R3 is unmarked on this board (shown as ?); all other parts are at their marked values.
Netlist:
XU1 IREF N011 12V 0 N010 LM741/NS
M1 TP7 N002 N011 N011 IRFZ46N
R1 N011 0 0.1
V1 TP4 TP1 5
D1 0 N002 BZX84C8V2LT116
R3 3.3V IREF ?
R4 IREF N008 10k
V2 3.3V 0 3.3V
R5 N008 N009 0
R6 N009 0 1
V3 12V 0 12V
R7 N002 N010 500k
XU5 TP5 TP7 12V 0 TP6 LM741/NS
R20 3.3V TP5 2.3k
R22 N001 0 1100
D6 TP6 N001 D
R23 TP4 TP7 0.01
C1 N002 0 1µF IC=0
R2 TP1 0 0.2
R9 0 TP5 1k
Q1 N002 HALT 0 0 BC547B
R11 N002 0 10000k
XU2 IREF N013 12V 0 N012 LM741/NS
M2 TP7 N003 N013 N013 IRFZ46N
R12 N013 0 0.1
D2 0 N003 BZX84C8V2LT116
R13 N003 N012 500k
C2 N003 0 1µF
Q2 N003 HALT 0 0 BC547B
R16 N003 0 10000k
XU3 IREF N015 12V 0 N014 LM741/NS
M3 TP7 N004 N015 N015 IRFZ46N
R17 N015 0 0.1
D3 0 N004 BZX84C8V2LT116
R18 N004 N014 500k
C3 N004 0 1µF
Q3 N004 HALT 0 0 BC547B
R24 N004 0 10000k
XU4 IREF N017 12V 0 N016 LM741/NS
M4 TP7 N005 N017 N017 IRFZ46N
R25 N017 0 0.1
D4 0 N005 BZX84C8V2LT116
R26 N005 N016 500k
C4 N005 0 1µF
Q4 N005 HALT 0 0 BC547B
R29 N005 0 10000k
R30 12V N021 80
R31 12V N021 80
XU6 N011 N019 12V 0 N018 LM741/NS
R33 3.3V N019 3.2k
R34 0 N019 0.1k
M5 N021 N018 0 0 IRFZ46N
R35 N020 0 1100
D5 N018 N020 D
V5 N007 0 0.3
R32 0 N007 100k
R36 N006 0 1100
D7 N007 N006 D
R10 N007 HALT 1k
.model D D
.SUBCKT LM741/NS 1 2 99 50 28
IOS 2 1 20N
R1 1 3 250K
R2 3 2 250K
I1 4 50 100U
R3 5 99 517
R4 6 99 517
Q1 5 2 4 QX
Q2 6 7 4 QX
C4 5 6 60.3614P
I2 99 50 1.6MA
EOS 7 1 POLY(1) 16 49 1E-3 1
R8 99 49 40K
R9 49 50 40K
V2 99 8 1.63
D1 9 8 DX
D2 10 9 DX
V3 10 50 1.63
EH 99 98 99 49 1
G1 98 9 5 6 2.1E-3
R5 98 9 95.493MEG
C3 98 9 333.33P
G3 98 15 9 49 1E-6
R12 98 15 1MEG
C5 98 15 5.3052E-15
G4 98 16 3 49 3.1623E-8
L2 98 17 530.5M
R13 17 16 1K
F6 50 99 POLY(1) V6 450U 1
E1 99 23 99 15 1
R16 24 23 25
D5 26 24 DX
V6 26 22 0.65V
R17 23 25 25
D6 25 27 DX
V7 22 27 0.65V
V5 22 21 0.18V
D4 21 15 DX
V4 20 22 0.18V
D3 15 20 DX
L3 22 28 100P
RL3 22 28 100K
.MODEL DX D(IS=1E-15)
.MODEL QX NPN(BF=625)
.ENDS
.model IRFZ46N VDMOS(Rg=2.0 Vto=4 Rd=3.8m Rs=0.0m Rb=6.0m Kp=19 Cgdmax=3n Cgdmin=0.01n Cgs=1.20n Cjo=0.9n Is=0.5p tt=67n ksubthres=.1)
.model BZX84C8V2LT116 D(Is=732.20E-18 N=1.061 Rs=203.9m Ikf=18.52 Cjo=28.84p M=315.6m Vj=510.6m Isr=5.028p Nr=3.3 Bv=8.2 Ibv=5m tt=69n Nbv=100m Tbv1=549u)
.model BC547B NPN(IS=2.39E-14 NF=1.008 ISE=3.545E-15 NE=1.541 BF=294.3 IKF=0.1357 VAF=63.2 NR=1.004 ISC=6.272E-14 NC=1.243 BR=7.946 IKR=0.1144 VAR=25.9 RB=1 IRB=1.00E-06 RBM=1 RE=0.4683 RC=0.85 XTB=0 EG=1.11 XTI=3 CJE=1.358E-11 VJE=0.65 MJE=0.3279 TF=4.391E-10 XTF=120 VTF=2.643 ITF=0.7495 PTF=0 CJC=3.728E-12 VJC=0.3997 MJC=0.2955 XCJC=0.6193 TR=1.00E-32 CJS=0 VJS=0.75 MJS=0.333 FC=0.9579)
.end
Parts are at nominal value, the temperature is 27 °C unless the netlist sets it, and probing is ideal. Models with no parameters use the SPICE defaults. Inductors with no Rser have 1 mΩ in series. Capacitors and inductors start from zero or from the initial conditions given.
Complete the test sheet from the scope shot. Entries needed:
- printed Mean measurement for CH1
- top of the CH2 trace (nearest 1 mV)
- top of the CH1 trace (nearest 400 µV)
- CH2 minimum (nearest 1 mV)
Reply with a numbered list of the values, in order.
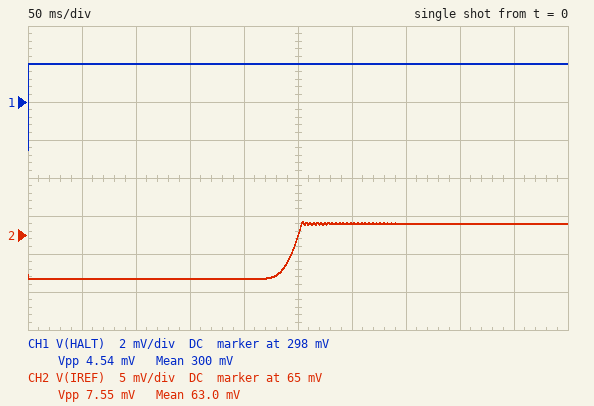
1. 300 mV
2. 67 mV
3. 300.0 mV
4. 59 mV
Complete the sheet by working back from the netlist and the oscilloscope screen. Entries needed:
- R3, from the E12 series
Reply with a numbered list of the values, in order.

1. 470 kΩ
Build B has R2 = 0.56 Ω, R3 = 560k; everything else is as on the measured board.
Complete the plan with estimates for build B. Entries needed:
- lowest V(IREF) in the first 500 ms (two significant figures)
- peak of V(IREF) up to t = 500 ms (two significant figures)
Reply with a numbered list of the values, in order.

1. 49 mV
2. 56 mV
